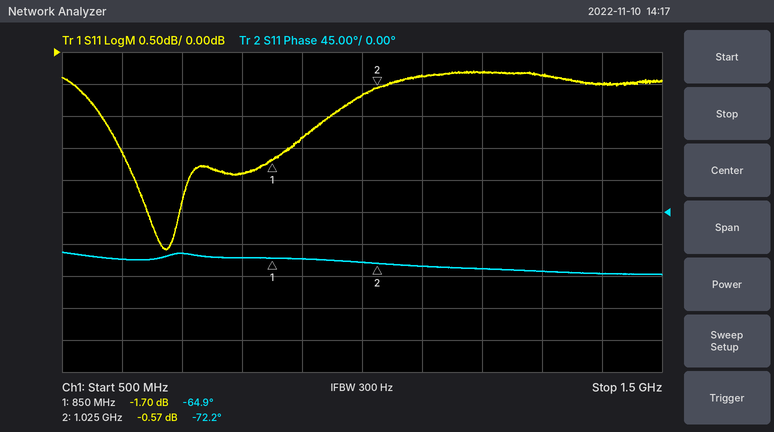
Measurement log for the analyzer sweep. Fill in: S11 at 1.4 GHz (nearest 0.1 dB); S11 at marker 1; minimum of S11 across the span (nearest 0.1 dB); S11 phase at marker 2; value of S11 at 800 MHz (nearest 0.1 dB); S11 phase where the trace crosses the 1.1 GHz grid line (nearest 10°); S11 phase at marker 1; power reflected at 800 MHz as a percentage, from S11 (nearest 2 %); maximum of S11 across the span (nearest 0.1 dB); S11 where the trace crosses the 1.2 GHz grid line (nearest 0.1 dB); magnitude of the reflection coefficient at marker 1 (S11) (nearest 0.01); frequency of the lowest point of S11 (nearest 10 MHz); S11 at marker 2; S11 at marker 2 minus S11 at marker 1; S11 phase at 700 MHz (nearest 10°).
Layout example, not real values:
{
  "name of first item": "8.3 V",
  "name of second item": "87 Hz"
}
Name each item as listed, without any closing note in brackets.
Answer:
{
  "S11 at 1.4 GHz": "-0.5 dB",
  "S11 at marker 1": "-1.70 dB",
  "minimum of S11 across the span": "-3.1 dB",
  "S11 phase at marker 2": "-72.2°",
  "value of S11 at 800 MHz": "-1.9 dB",
  "S11 phase where the trace crosses the 1.1 GHz grid line": "-80°",
  "S11 phase at marker 1": "-64.9°",
  "power reflected at 800 MHz as a percentage, from S11": "64 %",
  "maximum of S11 across the span": "-0.3 dB",
  "S11 where the trace crosses the 1.2 GHz grid line": "-0.3 dB",
  "magnitude of the reflection coefficient at marker 1 (S11)": "0.82",
  "frequency of the lowest point of S11": "670 MHz",
  "S11 at marker 2": "-0.57 dB",
  "S11 at marker 2 minus S11 at marker 1": "1.13 dB",
  "S11 phase at 700 MHz": "-60°"
}
